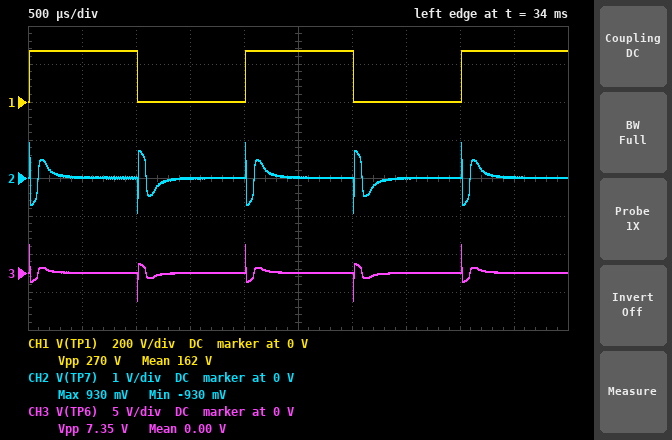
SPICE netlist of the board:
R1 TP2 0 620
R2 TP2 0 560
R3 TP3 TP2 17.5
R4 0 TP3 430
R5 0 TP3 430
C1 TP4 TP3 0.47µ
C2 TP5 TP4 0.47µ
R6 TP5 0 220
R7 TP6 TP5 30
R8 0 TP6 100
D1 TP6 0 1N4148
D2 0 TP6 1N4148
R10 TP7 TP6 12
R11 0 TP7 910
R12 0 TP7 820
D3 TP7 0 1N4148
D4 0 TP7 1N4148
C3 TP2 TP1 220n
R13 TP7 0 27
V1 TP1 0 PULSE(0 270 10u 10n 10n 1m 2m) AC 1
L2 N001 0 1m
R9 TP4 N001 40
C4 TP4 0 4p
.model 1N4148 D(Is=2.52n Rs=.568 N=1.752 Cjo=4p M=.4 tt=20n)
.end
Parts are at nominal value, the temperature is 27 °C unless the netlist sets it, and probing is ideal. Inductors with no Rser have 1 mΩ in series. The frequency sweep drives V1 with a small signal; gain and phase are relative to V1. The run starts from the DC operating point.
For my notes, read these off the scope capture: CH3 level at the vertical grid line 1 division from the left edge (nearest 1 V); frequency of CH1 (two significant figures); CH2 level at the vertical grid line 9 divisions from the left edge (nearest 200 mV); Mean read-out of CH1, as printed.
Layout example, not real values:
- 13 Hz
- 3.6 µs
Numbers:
- 0 V
- 500 Hz
- 0 V
- 162 V
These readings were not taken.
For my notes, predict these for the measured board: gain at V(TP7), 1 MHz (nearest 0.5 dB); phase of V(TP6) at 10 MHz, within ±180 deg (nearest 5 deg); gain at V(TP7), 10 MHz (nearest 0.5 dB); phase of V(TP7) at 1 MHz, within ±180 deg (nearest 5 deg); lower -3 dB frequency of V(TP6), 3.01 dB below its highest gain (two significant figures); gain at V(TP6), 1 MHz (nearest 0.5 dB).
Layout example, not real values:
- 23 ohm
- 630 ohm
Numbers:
- -13.0 dB
- 0 deg
- -13.0 dB
- 0 deg
- 22 kHz
- -10.0 dB
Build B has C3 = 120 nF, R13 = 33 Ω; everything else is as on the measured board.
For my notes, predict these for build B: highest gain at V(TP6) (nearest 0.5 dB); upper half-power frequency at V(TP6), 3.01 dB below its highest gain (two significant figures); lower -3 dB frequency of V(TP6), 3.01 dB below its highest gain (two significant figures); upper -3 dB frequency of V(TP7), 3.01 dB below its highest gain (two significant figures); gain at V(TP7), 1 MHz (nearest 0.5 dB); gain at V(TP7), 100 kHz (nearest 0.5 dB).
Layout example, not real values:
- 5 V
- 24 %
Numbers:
- -9.5 dB
- 630 MHz
- 33 kHz
- 590 MHz
- -12.0 dB
- -12.5 dB
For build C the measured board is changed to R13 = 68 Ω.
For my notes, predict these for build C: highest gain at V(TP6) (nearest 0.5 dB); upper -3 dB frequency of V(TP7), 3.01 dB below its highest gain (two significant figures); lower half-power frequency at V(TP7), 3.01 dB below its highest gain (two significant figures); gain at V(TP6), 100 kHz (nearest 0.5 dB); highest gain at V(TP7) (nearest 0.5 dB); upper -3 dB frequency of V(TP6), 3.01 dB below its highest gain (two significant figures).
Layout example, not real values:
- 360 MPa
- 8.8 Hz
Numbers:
- -7.5 dB
- 450 MHz
- 19 kHz
- -8.0 dB
- -9.5 dB
- 480 MHz
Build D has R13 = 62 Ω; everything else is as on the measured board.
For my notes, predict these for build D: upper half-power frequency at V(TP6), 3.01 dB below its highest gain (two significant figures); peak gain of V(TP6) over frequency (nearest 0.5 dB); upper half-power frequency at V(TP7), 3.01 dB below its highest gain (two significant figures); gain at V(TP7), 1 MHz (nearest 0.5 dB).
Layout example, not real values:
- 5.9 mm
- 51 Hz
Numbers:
- 490 MHz
- -8.0 dB
- 470 MHz
- -9.5 dB
